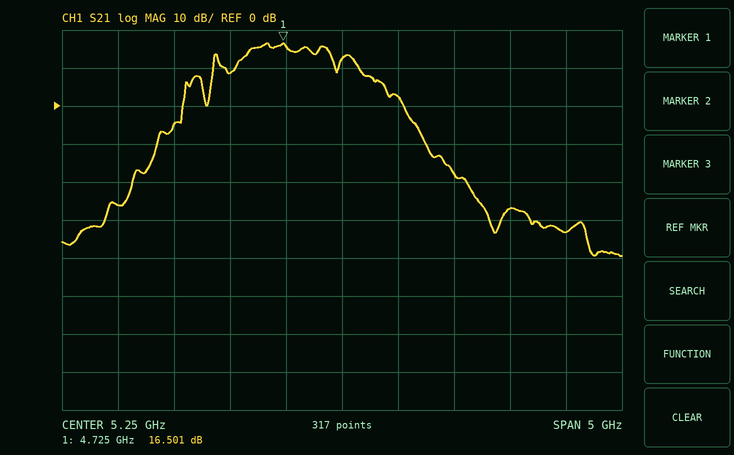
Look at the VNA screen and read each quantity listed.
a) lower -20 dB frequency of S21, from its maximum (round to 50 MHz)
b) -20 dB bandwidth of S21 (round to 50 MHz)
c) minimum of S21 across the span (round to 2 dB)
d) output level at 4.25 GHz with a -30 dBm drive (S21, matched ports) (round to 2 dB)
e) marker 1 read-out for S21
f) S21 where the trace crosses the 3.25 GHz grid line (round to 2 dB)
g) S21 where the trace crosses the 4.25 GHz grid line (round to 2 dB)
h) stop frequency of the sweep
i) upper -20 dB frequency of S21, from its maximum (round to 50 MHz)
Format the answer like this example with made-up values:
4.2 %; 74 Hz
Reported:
3.80 GHz; 2.05 GHz; -40 dB; -22 dBm; 16.501 dB; -26 dB; 8 dB; 7.75 GHz; 5.85 GHz
